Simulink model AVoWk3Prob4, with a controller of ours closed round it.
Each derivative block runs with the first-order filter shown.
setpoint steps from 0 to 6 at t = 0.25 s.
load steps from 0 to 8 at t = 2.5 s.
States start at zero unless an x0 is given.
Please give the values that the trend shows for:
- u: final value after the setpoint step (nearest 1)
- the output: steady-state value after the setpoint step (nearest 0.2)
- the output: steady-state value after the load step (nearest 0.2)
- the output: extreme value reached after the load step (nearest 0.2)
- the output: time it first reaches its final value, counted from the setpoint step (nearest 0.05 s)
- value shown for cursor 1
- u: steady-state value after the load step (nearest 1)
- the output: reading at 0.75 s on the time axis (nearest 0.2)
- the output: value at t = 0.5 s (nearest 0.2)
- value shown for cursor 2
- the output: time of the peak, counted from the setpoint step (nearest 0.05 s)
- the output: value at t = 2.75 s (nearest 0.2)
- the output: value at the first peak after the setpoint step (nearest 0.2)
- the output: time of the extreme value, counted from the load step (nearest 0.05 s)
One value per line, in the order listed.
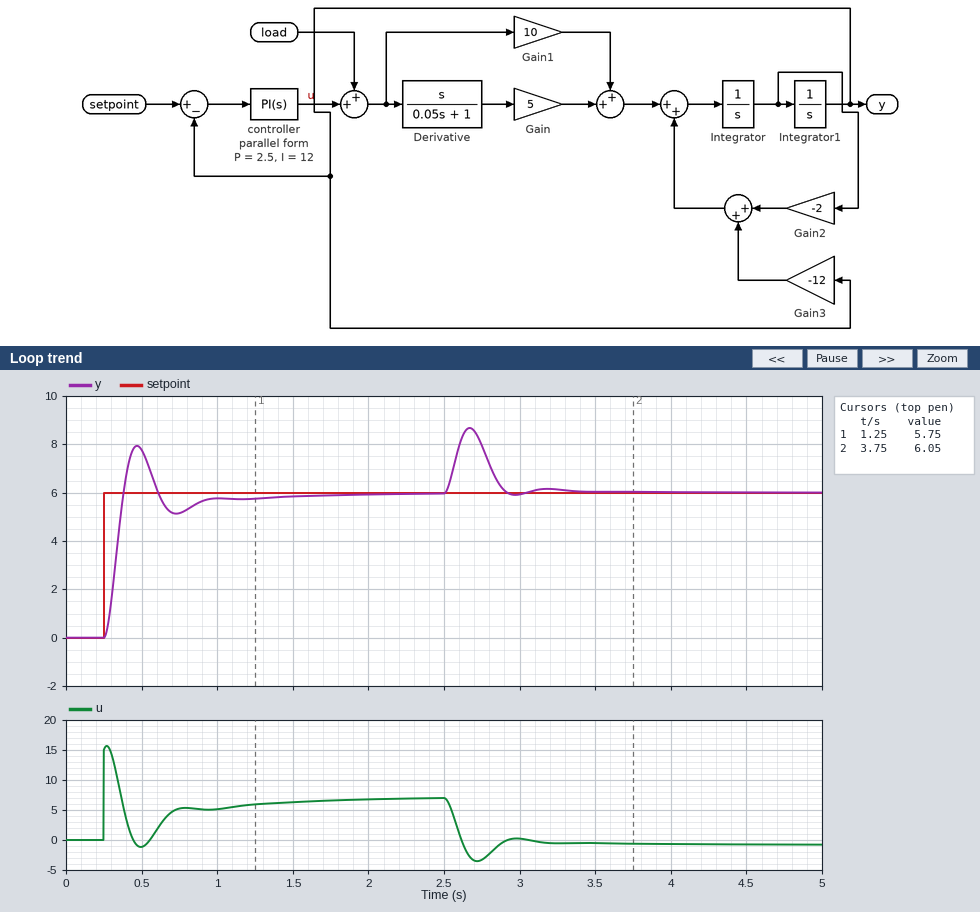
7
6.0
6.0
8.6
0.15 s
5.75
-1
5.2
7.8
6.05
0.20 s
8.0
8.0
0.15 s
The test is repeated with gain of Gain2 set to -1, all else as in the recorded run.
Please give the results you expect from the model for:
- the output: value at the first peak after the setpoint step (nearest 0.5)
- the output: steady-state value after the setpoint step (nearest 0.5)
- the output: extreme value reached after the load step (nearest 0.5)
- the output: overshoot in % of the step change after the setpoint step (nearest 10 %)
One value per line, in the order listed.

8.5
6.0
9.0
40 %
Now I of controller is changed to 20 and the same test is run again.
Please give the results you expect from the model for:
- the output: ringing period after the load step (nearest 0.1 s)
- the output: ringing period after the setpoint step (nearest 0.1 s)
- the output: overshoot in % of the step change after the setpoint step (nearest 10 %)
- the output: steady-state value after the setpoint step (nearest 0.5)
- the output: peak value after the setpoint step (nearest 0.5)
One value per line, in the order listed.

0.5 s
0.5 s
50 %
6.0
9.0
